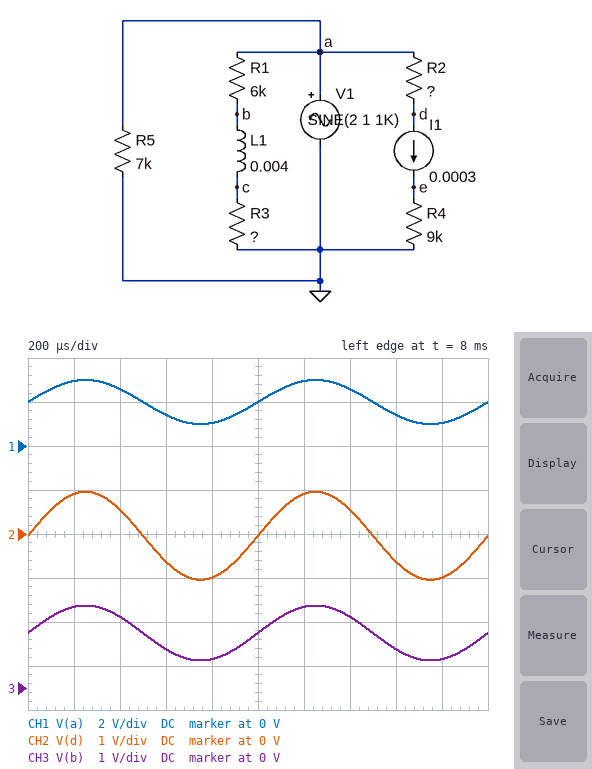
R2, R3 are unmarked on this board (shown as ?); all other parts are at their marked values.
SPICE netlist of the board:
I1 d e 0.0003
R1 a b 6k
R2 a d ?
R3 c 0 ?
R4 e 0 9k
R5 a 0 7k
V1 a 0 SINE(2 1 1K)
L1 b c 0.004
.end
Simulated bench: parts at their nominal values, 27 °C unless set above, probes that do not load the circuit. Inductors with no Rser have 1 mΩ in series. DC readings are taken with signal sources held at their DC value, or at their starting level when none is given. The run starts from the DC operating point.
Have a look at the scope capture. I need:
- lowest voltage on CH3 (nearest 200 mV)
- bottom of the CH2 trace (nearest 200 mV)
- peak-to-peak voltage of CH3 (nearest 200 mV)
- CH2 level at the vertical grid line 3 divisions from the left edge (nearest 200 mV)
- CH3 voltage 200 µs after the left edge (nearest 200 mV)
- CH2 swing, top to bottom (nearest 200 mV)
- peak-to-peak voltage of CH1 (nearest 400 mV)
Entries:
600 mV
-1.0 V
1.2 V
-600 mV
1.8 V
2.0 V
2.0 V
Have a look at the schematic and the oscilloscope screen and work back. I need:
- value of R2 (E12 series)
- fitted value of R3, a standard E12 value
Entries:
6.8 kΩ
10 kΩ
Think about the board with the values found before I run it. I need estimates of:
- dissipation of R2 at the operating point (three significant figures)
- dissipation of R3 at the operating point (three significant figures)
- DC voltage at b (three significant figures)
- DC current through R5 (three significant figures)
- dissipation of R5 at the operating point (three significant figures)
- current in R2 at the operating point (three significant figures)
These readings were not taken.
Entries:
612 µW
156 µW
1.25 V
286 µA
571 µW
300 µA
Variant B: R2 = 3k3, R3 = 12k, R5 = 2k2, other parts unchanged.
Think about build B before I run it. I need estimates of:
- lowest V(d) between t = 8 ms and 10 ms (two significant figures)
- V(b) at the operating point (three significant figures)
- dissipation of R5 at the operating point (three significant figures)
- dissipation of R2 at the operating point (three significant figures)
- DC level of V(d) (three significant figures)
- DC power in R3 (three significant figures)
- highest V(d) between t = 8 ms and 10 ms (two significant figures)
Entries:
10 mV
1.33 V
1.82 mW
297 µW
1.01 V
148 µW
2.0 V
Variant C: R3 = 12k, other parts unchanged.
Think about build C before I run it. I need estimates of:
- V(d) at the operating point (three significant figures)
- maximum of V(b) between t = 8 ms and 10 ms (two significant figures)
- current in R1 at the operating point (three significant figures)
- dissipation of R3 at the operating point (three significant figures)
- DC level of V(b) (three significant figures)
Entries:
-40.0 mV
2.0 V
111 µA
148 µW
1.33 V
